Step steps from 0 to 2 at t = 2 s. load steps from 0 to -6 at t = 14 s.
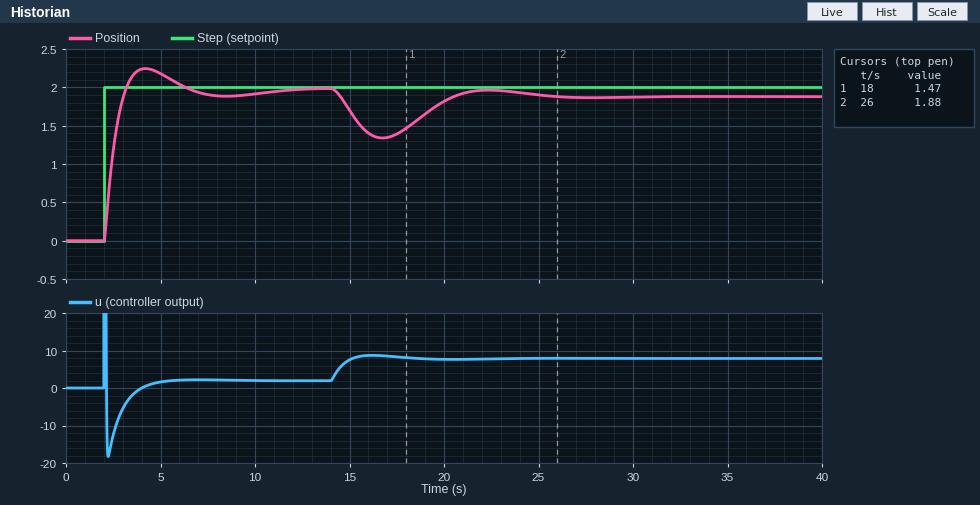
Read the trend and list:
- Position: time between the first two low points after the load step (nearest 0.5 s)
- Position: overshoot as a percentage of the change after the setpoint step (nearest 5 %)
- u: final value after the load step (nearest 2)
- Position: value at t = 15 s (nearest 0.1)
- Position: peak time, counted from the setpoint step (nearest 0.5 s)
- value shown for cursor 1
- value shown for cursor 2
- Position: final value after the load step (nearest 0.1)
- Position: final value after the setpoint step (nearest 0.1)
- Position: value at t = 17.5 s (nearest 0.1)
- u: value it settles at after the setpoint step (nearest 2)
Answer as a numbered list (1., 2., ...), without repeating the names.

1. 11.0 s
2. 15 %
3. 8
4. 1.7
5. 2.0 s
6. 1.47
7. 1.88
8. 1.9
9. 2.0
10. 1.4
11. 2
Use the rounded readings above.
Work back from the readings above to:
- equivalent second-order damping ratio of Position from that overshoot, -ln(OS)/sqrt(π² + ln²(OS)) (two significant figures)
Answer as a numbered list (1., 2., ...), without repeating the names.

1. 0.52
